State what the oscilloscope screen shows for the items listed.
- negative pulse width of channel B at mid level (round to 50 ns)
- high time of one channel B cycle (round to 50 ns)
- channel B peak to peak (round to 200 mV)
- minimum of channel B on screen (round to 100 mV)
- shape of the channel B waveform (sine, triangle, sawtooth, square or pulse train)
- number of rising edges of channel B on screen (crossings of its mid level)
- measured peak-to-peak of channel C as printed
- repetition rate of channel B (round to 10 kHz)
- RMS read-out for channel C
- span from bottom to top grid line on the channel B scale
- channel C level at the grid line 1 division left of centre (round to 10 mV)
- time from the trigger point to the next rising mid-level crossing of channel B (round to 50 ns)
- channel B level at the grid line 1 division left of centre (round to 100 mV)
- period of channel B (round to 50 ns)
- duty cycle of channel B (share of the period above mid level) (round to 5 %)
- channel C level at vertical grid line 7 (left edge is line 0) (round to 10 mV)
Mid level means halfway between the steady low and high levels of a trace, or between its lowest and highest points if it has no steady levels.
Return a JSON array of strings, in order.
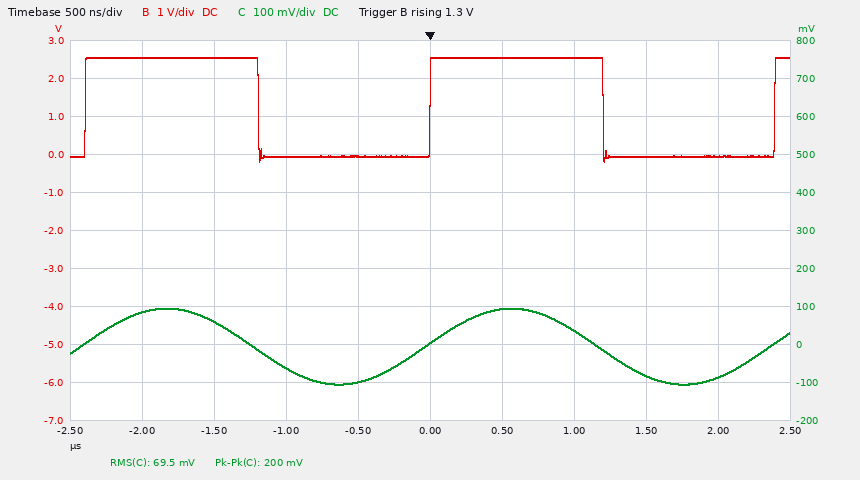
["1.20 µs", "1.20 µs", "2.8 V", "-200 mV", "square", "3", "200 mV", "420 kHz", "69.5 mV", "10 V", "-100 mV", "2.40 µs", "0.0 V", "2.40 µs", "50 %", "40 mV"]
